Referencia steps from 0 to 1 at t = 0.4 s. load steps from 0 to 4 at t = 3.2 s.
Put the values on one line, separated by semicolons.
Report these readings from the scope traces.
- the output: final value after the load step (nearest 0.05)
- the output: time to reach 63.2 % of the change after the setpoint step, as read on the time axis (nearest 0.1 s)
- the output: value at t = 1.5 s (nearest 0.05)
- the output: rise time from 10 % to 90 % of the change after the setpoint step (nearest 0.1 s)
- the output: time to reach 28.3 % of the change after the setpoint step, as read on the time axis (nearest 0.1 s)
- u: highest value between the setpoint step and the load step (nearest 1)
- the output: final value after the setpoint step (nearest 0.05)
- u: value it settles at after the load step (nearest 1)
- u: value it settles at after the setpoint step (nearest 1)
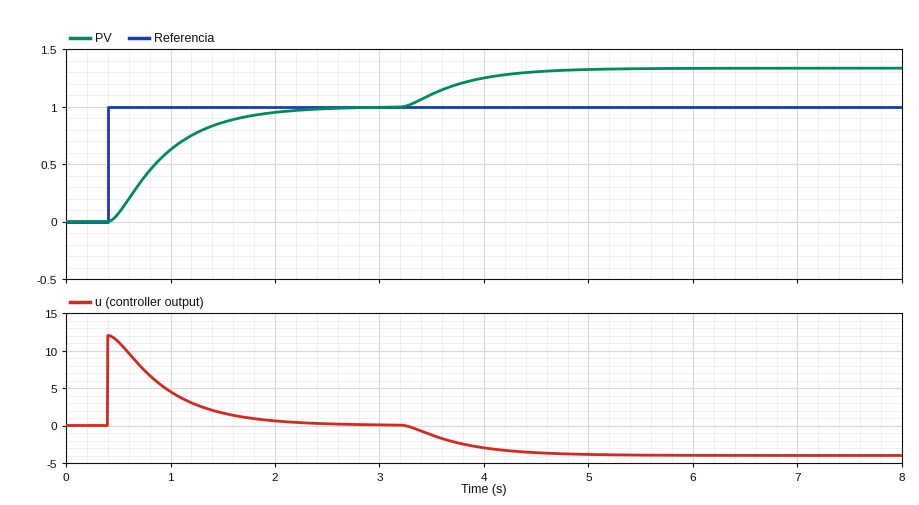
1.35; 1.0 s; 0.85; 1.1 s; 0.7 s; 12; 1.00; -4; 0
